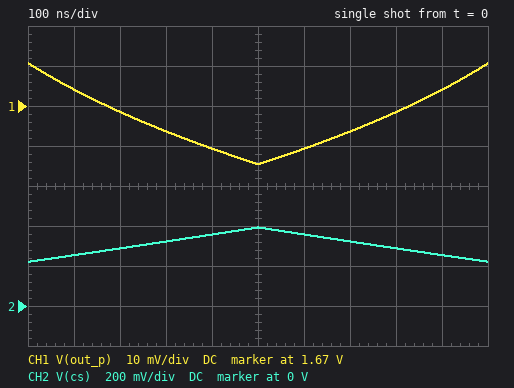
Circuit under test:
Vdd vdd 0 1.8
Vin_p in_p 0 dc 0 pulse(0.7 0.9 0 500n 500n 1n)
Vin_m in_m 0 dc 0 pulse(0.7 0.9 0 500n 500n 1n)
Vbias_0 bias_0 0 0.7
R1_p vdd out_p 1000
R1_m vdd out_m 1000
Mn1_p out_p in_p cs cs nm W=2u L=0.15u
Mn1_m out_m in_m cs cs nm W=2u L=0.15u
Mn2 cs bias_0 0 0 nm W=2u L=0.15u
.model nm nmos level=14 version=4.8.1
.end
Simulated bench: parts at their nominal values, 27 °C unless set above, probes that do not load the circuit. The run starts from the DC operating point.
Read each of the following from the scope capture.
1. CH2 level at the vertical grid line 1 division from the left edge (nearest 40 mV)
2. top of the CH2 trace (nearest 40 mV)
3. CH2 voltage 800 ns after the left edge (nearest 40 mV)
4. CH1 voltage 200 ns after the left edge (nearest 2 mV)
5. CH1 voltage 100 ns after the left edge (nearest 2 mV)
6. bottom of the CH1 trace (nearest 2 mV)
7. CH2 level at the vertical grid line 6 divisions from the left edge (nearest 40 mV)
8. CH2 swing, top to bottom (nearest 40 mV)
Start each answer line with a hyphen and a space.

- 240 mV
- 400 mV
- 280 mV
- 1.668 V
- 1.674 V
- 1.656 V
- 360 mV
- 160 mV
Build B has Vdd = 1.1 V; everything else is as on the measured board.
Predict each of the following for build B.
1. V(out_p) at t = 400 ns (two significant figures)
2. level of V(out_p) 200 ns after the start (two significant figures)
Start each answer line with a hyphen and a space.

- 960 mV
- 970 mV
